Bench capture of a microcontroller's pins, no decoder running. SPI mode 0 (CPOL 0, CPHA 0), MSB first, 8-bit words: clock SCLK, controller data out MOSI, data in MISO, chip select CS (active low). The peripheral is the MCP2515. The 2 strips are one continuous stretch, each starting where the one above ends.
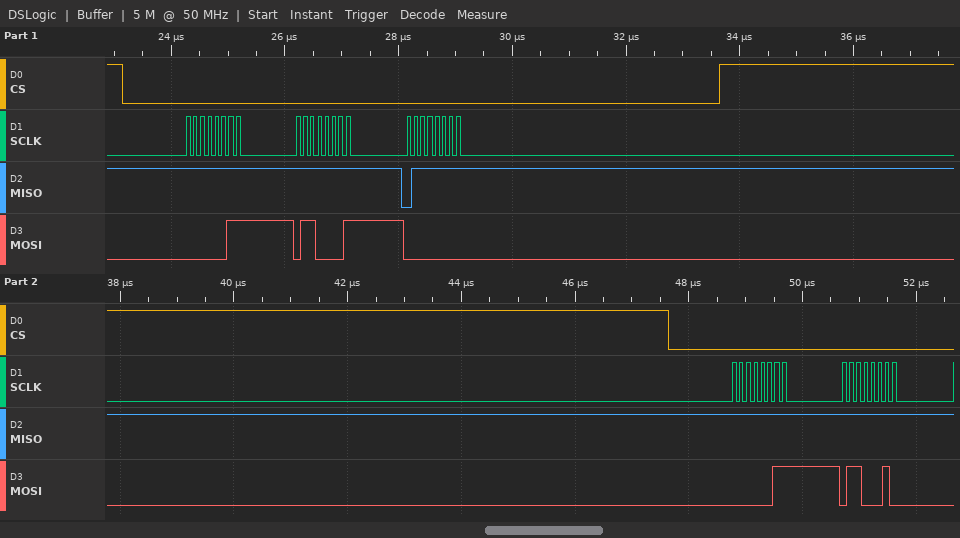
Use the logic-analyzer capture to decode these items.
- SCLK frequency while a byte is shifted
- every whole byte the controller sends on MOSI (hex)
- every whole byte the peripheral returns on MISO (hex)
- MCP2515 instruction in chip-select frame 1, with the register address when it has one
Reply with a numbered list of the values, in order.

1. 8 MHz
2. 0x03 0x61 0x00 0x03 0x62
3. 0xFF 0xFF 0x7F 0xFF 0xFF
4. READ 0x61
